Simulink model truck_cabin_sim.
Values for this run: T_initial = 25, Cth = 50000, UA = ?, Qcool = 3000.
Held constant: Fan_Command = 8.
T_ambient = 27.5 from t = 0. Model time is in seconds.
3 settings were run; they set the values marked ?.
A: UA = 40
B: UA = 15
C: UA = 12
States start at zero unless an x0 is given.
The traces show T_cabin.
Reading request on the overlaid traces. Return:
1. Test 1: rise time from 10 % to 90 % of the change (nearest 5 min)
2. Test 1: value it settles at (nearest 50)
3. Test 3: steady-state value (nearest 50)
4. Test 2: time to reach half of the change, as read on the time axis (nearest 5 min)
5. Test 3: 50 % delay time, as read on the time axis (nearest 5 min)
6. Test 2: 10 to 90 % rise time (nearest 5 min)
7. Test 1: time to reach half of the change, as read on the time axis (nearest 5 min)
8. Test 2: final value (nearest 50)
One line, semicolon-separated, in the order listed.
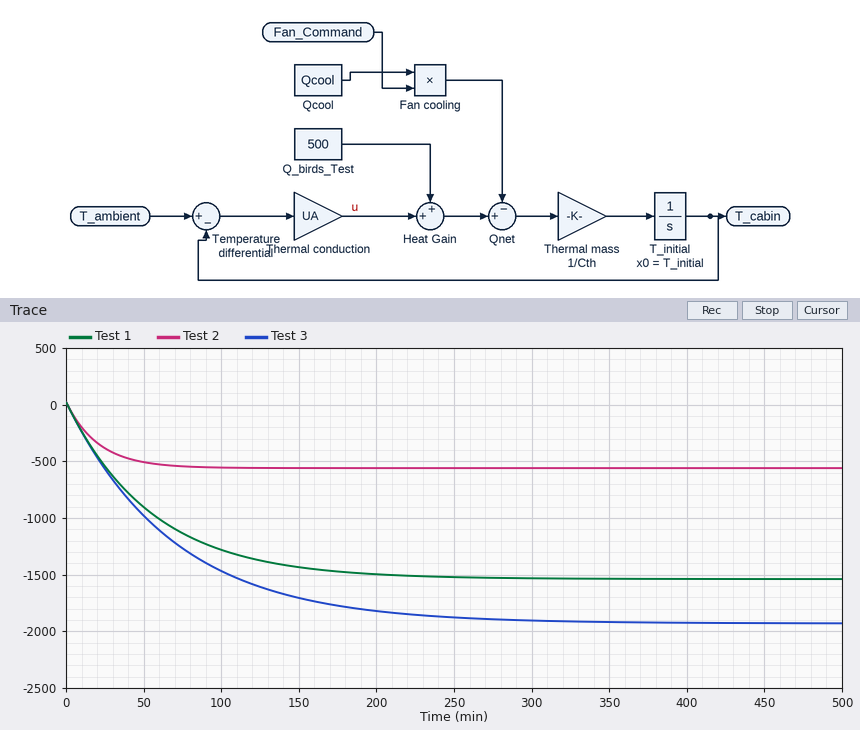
120 min; -1550; -1950; 15 min; 50 min; 45 min; 40 min; -550
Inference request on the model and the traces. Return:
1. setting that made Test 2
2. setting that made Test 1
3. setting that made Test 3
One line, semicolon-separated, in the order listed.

A; B; C
